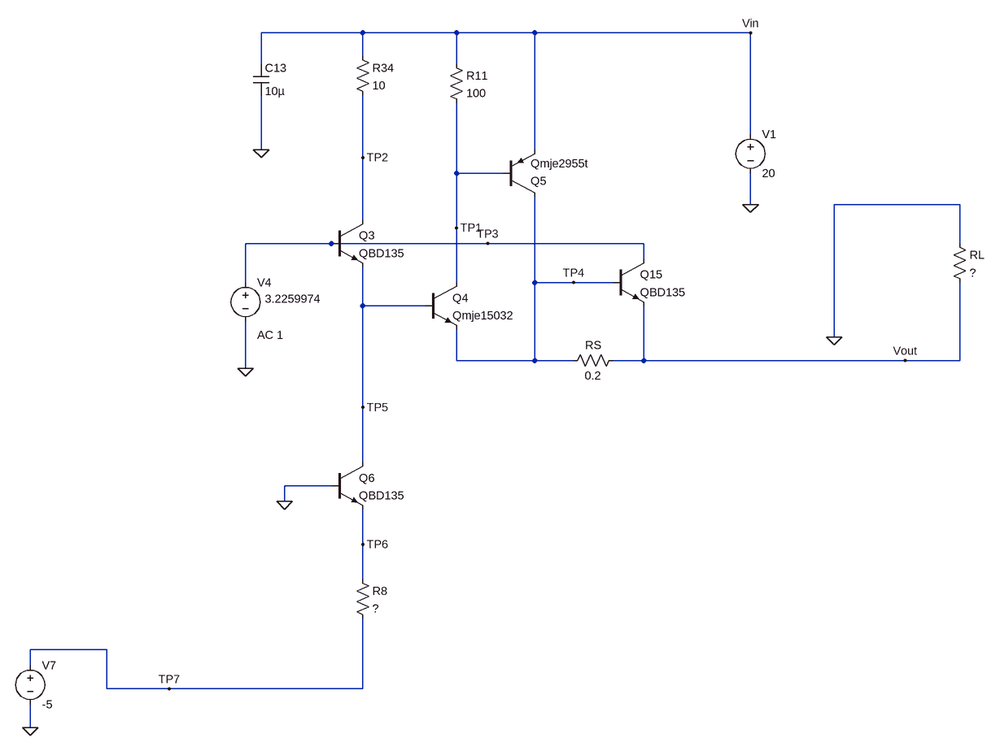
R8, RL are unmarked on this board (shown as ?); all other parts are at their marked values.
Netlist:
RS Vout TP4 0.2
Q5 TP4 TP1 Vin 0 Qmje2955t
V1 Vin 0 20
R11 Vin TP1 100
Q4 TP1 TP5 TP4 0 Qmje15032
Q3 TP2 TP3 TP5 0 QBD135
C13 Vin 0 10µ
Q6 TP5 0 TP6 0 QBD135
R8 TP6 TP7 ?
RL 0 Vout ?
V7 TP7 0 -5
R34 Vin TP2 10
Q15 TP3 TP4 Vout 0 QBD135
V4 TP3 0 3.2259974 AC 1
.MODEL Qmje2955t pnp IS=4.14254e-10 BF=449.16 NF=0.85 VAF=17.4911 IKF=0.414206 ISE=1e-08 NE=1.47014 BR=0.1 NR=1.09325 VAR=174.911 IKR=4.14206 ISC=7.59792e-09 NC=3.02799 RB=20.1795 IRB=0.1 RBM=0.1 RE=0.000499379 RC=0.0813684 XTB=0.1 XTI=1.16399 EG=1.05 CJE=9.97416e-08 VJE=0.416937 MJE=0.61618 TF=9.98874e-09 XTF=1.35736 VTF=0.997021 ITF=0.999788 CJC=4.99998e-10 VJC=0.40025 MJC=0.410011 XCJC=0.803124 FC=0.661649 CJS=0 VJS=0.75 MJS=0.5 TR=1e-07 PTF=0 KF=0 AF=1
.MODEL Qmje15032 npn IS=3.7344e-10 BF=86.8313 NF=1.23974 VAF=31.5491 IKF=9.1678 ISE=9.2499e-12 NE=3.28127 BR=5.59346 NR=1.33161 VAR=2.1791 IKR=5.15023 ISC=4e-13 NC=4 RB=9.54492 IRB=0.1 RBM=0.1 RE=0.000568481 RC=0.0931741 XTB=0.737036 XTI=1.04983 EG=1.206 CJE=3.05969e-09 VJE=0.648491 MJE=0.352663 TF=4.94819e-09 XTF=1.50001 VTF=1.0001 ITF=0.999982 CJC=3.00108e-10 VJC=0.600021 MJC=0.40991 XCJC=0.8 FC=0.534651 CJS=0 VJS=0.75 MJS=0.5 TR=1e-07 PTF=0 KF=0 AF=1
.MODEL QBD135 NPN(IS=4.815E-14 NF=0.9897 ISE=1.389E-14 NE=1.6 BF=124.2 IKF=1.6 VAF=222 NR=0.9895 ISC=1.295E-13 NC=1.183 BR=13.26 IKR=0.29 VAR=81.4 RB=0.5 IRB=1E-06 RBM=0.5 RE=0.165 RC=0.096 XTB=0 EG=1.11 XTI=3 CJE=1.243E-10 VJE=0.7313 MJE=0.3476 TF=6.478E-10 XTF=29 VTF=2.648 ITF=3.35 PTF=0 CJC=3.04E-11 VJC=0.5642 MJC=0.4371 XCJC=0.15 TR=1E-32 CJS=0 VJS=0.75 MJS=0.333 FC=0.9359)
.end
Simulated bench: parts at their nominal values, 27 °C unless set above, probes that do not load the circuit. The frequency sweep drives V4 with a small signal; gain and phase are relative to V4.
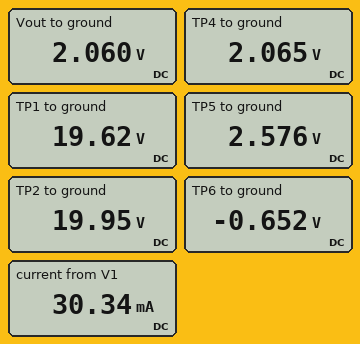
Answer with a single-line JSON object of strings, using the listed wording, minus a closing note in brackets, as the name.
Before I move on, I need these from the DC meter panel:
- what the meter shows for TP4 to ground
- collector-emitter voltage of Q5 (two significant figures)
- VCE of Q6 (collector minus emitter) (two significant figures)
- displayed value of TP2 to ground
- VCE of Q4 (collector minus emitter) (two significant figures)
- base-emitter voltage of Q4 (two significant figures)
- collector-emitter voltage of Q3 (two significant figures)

{"what the meter shows for TP4 to ground": "2.065 V", "collector-emitter voltage of Q5": "-18 V", "VCE of Q6 (collector minus emitter)": "3.2 V", "displayed value of TP2 to ground": "19.95 V", "VCE of Q4 (collector minus emitter)": "18 V", "base-emitter voltage of Q4": "510 mV", "collector-emitter voltage of Q3": "17 V"}
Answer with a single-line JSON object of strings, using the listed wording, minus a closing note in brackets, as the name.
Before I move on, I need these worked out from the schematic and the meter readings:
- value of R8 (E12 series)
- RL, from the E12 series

{"value of R8": "820 Ω", "RL, from the E12 series": "82 Ω"}
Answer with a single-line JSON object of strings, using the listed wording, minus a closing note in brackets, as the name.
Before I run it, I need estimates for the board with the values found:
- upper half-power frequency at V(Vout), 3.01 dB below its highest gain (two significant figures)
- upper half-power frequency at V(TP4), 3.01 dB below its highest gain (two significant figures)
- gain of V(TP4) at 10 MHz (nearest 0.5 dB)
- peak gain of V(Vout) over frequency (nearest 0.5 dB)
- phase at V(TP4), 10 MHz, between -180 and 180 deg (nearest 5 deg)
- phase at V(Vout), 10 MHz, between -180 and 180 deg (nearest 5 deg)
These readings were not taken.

{"upper half-power frequency at V(Vout), 3.01 dB below its highest gain": "33 MHz", "upper half-power frequency at V(TP4), 3.01 dB below its highest gain": "33 MHz", "gain of V(TP4) at 10 MHz": "-1.5 dB", "peak gain of V(Vout) over frequency": "0 dB", "phase at V(TP4), 10 MHz, between -180 and 180 deg": "-10 deg", "phase at V(Vout), 10 MHz, between -180 and 180 deg": "-10 deg"}
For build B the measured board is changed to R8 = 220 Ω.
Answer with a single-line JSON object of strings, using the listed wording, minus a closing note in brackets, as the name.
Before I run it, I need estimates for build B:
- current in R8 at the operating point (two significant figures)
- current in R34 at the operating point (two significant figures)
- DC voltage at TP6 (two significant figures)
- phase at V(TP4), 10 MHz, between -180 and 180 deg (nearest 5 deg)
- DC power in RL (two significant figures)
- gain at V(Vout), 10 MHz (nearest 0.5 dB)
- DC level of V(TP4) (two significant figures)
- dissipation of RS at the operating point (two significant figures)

{"current in R8 at the operating point": "20 mA", "current in R34 at the operating point": "19 mA", "DC voltage at TP6": "-690 mV", "phase at V(TP4), 10 MHz, between -180 and 180 deg": "-5 deg", "DC power in RL": "50 mW", "gain at V(Vout), 10 MHz": "-1.5 dB", "DC level of V(TP4)": "2.0 V", "dissipation of RS at the operating point": "120 µW"}
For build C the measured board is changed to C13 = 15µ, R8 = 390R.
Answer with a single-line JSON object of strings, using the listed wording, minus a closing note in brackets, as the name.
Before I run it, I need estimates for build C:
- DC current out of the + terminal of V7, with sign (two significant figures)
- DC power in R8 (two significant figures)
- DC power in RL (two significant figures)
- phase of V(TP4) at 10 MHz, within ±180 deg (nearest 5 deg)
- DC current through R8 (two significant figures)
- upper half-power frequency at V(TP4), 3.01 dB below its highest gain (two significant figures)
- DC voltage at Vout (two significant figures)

{"DC current out of the + terminal of V7, with sign": "-11 mA", "DC power in R8": "48 mW", "DC power in RL": "51 mW", "phase of V(TP4) at 10 MHz, within ±180 deg": "-5 deg", "DC current through R8": "11 mA", "upper half-power frequency at V(TP4), 3.01 dB below its highest gain": "44 MHz", "DC voltage at Vout": "2.0 V"}
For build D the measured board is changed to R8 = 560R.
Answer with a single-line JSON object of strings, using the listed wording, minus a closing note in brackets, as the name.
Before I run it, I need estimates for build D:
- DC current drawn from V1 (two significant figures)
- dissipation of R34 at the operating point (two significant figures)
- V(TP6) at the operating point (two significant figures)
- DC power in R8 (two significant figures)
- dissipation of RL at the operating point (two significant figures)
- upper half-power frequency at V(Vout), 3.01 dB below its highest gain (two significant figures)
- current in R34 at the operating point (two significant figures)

{"DC current drawn from V1": "33 mA", "dissipation of R34 at the operating point": "590 µW", "V(TP6) at the operating point": "-660 mV", "DC power in R8": "34 mW", "dissipation of RL at the operating point": "51 mW", "upper half-power frequency at V(Vout), 3.01 dB below its highest gain": "39 MHz", "current in R34 at the operating point": "7.7 mA"}
